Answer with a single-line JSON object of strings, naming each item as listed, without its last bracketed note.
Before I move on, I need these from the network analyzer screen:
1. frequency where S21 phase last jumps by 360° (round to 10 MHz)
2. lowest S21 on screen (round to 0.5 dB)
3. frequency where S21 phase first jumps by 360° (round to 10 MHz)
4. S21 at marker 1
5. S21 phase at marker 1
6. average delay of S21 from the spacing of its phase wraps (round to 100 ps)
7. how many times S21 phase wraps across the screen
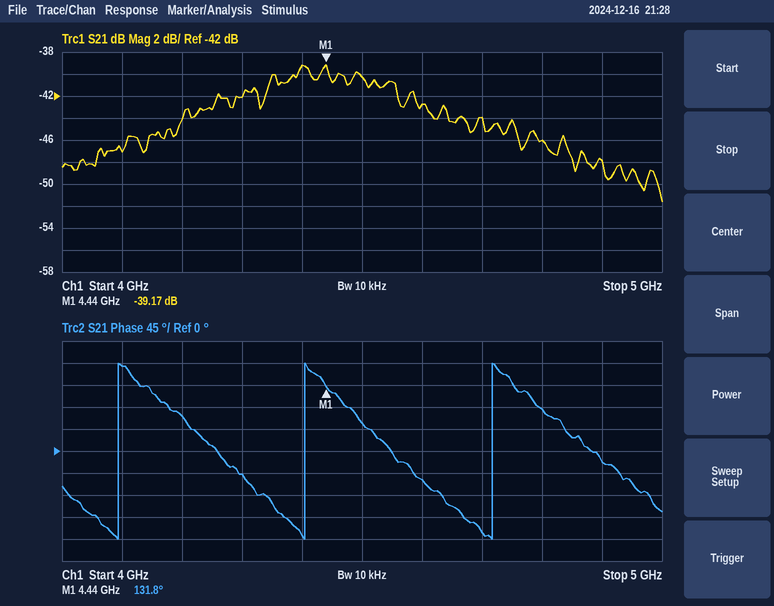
{"frequency where S21 phase last jumps by 360°": "4.72 GHz", "lowest S21 on screen": "-51.5 dB", "frequency where S21 phase first jumps by 360°": "4.09 GHz", "S21 at marker 1": "-39.17 dB", "S21 phase at marker 1": "131.8°", "average delay of S21 from the spacing of its phase wraps": "3.2 ns", "how many times S21 phase wraps across the screen": "3"}
